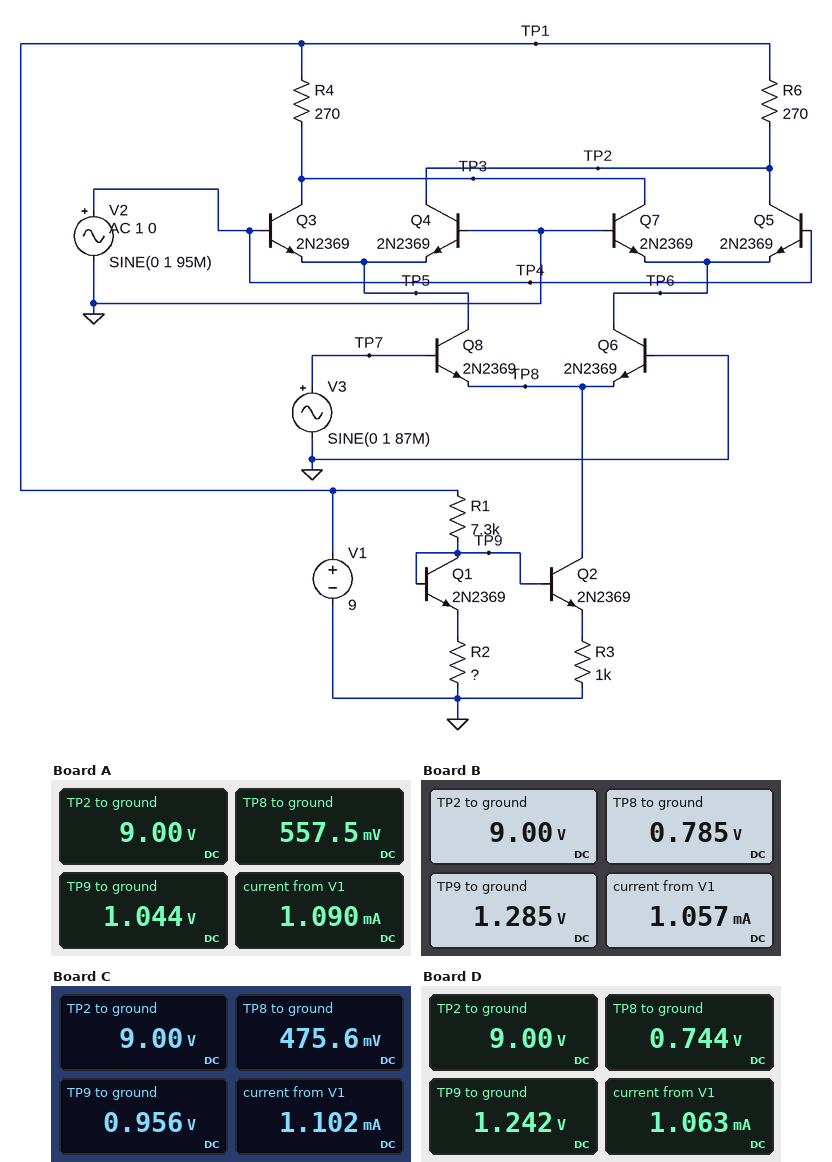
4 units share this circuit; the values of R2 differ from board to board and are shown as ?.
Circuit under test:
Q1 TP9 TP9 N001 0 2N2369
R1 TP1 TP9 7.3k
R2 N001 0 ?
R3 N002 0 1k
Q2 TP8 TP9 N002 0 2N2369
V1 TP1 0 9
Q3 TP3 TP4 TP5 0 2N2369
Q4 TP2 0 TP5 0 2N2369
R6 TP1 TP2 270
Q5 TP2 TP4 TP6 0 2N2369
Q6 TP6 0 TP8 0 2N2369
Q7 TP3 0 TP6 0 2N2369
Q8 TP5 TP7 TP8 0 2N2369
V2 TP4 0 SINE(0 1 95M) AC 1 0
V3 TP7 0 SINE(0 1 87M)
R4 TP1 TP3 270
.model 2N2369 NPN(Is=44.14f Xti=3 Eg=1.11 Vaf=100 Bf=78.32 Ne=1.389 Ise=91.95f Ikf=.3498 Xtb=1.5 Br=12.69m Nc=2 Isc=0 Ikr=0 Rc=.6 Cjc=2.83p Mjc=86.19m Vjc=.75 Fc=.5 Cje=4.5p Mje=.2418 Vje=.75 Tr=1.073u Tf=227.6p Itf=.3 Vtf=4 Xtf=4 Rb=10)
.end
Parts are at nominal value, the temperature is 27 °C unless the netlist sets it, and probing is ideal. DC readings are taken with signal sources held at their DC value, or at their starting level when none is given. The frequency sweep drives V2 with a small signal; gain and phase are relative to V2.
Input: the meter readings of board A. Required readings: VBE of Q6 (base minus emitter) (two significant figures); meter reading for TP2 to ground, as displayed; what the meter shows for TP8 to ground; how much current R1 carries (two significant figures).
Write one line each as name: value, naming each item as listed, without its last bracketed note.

VBE of Q6 (base minus emitter): -560 mV
meter reading for TP2 to ground, as displayed: 9.00 V
what the meter shows for TP8 to ground: 557.5 mV
how much current R1 carries: 1.1 mA
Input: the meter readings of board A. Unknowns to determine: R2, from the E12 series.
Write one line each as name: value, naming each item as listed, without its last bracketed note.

R2, from the E12 series: 680 Ω
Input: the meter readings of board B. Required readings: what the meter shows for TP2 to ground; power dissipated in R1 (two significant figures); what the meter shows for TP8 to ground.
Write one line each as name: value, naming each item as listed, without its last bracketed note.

what the meter shows for TP2 to ground: 9.00 V
power dissipated in R1: 8.2 mW
what the meter shows for TP8 to ground: 0.785 V
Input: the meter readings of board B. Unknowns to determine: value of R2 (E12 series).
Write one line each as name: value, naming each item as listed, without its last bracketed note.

value of R2: 1.8 kΩ
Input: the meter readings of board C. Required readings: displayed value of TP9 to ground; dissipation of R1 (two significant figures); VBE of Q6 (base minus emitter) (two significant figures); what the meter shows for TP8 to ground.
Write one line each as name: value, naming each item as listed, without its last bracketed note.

displayed value of TP9 to ground: 0.956 V
dissipation of R1: 8.9 mW
VBE of Q6 (base minus emitter): -480 mV
what the meter shows for TP8 to ground: 475.6 mV
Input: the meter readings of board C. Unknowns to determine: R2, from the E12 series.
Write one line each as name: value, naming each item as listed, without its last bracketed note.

R2, from the E12 series: 470 Ω
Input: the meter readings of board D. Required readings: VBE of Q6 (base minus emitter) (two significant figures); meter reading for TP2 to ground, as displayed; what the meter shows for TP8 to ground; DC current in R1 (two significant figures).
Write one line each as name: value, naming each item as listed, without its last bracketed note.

VBE of Q6 (base minus emitter): -740 mV
meter reading for TP2 to ground, as displayed: 9.00 V
what the meter shows for TP8 to ground: 0.744 V
DC current in R1: 1.1 mA
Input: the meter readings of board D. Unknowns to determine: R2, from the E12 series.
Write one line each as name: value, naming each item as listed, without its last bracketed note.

R2, from the E12 series: 1.5 kΩ
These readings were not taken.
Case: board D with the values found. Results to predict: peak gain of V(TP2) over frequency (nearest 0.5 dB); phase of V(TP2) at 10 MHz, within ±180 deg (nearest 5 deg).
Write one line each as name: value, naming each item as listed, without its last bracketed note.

peak gain of V(TP2) over frequency: -6.5 dB
phase of V(TP2) at 10 MHz, within ±180 deg: 85 deg
